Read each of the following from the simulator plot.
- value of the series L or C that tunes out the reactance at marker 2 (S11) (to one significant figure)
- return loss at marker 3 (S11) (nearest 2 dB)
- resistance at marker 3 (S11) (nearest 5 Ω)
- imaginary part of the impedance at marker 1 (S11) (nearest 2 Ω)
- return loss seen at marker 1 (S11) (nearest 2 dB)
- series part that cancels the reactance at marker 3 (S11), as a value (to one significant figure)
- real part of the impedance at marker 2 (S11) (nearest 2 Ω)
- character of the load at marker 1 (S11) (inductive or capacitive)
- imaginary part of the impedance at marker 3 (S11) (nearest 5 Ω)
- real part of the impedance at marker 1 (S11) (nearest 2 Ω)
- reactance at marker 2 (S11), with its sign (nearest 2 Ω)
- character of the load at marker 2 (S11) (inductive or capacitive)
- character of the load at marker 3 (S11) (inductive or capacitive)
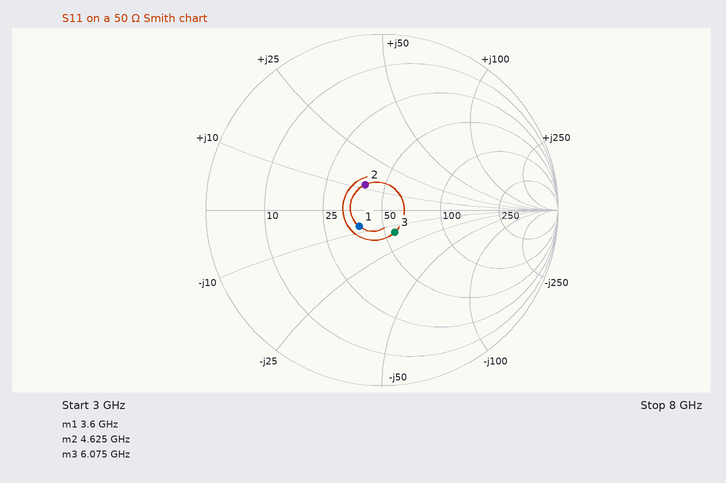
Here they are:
3 pF
16 dB
55 Ω
-8 Ω
16 dB
400 pH
40 Ω
capacitive
-15 Ω
38 Ω
+12 Ω
inductive
capacitive
